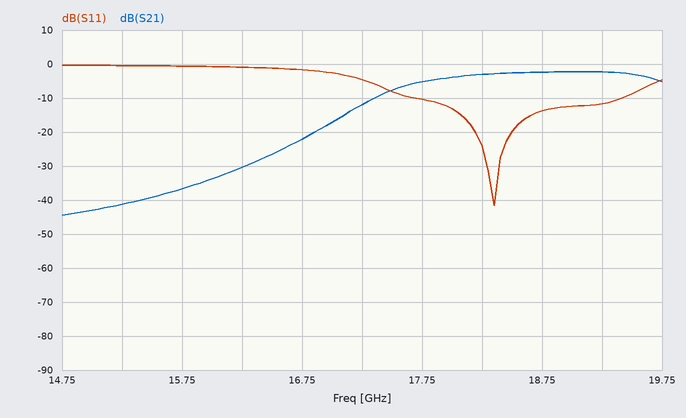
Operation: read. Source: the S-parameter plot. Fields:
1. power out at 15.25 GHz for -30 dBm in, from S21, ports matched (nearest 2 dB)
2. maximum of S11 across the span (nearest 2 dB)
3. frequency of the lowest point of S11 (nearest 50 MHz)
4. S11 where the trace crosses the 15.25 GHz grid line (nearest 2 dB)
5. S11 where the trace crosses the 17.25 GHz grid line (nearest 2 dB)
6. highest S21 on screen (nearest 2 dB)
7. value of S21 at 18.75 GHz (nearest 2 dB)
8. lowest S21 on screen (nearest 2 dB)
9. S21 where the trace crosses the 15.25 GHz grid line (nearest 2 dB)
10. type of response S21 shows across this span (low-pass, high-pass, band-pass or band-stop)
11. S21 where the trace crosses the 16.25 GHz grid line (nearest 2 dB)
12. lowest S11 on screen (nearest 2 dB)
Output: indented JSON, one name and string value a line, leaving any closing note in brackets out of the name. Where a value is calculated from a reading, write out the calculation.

{
  "power out at 15.25 GHz for -30 dBm in, from S21, ports matched": "-30 dBm + (-42 dB) = -72 dBm",
  "maximum of S11 across the span": "0 dB",
  "frequency of the lowest point of S11": "18.35 GHz",
  "S11 where the trace crosses the 15.25 GHz grid line": "0 dB",
  "S11 where the trace crosses the 17.25 GHz grid line": "-4 dB",
  "highest S21 on screen": "-2 dB",
  "value of S21 at 18.75 GHz": "-2 dB",
  "lowest S21 on screen": "-44 dB",
  "S21 where the trace crosses the 15.25 GHz grid line": "-42 dB",
  "type of response S21 shows across this span": "high-pass",
  "S21 where the trace crosses the 16.25 GHz grid line": "-30 dB",
  "lowest S11 on screen": "-42 dB"
}
